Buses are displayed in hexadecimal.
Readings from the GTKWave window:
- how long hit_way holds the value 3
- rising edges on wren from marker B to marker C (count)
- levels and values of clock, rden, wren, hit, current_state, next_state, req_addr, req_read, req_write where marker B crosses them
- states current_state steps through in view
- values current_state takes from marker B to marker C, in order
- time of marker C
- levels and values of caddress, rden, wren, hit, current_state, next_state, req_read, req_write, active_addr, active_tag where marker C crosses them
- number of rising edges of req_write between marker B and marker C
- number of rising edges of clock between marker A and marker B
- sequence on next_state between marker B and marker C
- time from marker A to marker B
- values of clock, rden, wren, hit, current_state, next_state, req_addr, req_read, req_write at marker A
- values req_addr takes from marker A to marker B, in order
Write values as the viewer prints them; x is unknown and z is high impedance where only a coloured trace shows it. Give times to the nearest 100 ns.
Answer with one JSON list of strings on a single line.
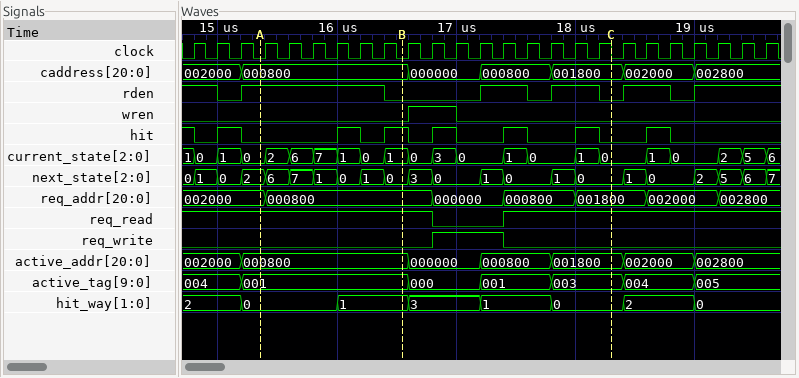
["600 ns", "1", "clock=0, rden=0, wren=0, hit=1, current_state=1, next_state=0, req_addr=000800, req_read=1, req_write=0", "1, 0, 1, 0, 2, 6, 7, 1, 0, 1, 0, 3, 0, 1, 0, 1, 0, 1, 0, 2, 5, 6", "1, 0, 3, 0, 1, 0, 1, 0", "18300 ns", "caddress=001800, rden=0, wren=0, hit=0, current_state=0, next_state=0, req_read=1, req_write=0, active_addr=001800, active_tag=003", "1", "6", "0, 3, 0, 1, 0, 1, 0", "1200 ns", "clock=0, rden=1, wren=0, hit=0, current_state=0, next_state=2, req_addr=002000, req_read=1, req_write=0", "002000, 000800"]
